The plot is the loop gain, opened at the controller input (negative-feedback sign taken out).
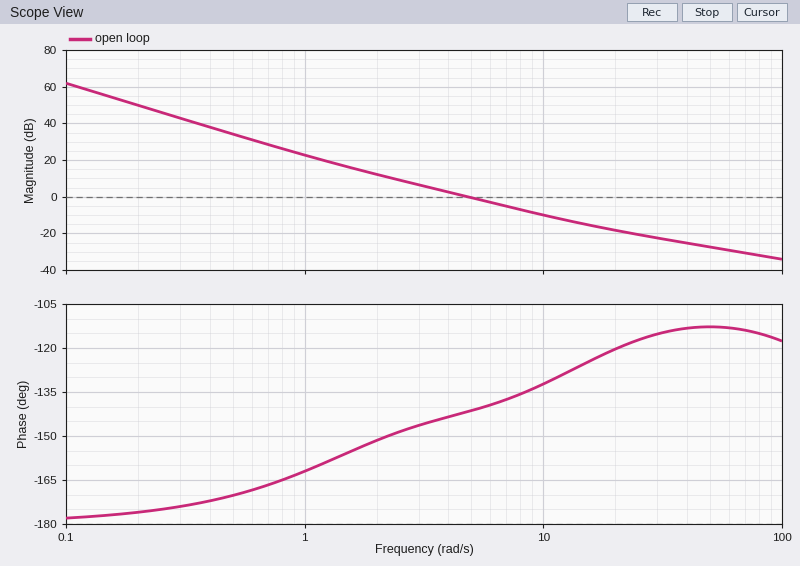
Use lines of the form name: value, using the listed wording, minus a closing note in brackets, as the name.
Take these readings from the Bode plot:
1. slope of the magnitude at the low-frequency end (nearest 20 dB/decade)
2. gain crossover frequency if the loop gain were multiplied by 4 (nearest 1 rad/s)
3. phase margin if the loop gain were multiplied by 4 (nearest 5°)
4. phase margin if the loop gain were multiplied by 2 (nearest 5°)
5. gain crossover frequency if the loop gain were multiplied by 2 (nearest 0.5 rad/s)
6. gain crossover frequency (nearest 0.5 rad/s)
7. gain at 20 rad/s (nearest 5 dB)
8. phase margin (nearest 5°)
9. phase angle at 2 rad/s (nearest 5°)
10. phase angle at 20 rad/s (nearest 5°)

slope of the magnitude at the low-frequency end: -40 dB/decade
gain crossover frequency if the loop gain were multiplied by 4: 12 rad/s
phase margin if the loop gain were multiplied by 4: 50°
phase margin if the loop gain were multiplied by 2: 45°
gain crossover frequency if the loop gain were multiplied by 2: 7.5 rad/s
gain crossover frequency: 5.0 rad/s
gain at 20 rad/s: -20 dB
phase margin: 40°
phase angle at 2 rad/s: -150°
phase angle at 20 rad/s: -120°
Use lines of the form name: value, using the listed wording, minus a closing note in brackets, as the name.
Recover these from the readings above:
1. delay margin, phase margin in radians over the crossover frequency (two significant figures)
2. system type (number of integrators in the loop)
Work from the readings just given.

delay margin, phase margin in radians over the crossover frequency: 0.14 s
system type: 2
